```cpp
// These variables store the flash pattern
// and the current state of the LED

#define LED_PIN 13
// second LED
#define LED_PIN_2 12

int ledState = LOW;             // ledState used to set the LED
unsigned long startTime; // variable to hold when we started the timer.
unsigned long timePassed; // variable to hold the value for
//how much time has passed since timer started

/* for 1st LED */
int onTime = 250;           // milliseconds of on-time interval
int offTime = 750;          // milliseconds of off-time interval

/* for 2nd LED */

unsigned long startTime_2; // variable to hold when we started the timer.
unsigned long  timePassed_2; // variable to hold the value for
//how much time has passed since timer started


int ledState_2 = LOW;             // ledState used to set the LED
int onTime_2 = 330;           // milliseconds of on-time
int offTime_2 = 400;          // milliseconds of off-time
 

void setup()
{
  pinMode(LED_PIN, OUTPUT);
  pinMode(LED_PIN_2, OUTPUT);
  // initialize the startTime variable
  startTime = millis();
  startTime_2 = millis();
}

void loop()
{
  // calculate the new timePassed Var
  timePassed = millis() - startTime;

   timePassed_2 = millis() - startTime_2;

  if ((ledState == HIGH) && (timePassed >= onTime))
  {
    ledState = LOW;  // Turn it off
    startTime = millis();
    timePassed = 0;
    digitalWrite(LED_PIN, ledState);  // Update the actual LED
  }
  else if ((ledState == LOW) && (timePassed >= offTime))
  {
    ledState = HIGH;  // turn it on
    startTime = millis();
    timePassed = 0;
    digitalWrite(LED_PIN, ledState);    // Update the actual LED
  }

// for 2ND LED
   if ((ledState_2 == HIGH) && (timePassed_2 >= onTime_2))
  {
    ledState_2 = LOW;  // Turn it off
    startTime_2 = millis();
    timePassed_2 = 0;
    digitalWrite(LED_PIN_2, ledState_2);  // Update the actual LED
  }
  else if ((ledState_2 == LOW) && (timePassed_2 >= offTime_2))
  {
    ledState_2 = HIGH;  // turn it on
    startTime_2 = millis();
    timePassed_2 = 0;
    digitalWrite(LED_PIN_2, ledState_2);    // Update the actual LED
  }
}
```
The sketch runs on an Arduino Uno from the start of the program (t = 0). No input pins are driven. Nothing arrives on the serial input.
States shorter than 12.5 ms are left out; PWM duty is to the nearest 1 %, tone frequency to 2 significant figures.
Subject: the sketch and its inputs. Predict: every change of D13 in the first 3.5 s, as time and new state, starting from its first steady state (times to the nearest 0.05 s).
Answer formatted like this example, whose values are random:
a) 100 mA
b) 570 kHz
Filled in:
a) 0 s low; 0.75 s high; 1 s low; 1.75 s high; 2 s low; 2.75 s high; 3 s low
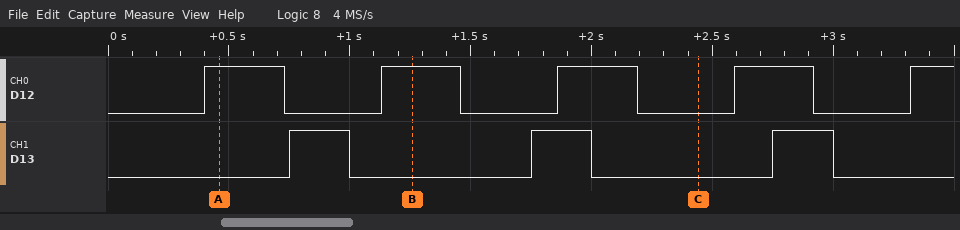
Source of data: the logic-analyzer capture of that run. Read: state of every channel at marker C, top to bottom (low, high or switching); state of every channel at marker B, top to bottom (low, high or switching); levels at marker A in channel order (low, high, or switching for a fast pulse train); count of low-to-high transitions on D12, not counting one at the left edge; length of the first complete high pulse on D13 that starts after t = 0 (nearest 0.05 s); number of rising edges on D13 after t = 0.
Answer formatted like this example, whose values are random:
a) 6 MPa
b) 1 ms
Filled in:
a) D12 low, D13 low
b) D12 high, D13 low
c) D12 high, D13 low
d) 5
e) 0.25 s
f) 3
